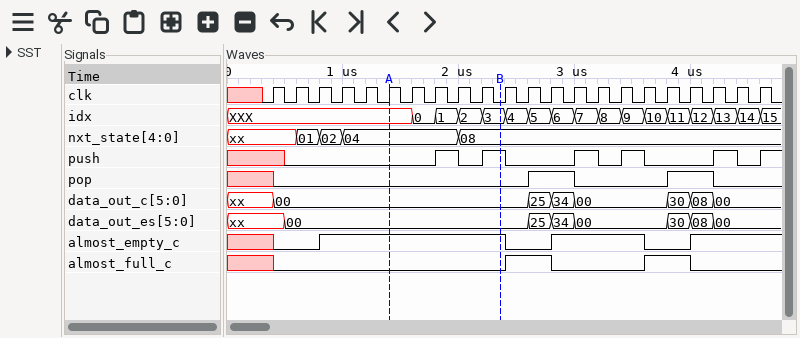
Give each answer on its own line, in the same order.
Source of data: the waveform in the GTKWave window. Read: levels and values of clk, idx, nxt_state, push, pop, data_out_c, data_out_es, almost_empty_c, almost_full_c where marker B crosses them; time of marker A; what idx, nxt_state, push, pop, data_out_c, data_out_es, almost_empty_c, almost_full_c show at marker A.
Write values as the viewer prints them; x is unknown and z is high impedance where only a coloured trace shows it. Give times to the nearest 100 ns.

clk=0, idx=3, nxt_state=08, push=1, pop=0, data_out_c=00, data_out_es=00, almost_empty_c=1, almost_full_c=0
1400 ns
idx=XXX, nxt_state=04, push=0, pop=0, data_out_c=00, data_out_es=00, almost_empty_c=1, almost_full_c=0
